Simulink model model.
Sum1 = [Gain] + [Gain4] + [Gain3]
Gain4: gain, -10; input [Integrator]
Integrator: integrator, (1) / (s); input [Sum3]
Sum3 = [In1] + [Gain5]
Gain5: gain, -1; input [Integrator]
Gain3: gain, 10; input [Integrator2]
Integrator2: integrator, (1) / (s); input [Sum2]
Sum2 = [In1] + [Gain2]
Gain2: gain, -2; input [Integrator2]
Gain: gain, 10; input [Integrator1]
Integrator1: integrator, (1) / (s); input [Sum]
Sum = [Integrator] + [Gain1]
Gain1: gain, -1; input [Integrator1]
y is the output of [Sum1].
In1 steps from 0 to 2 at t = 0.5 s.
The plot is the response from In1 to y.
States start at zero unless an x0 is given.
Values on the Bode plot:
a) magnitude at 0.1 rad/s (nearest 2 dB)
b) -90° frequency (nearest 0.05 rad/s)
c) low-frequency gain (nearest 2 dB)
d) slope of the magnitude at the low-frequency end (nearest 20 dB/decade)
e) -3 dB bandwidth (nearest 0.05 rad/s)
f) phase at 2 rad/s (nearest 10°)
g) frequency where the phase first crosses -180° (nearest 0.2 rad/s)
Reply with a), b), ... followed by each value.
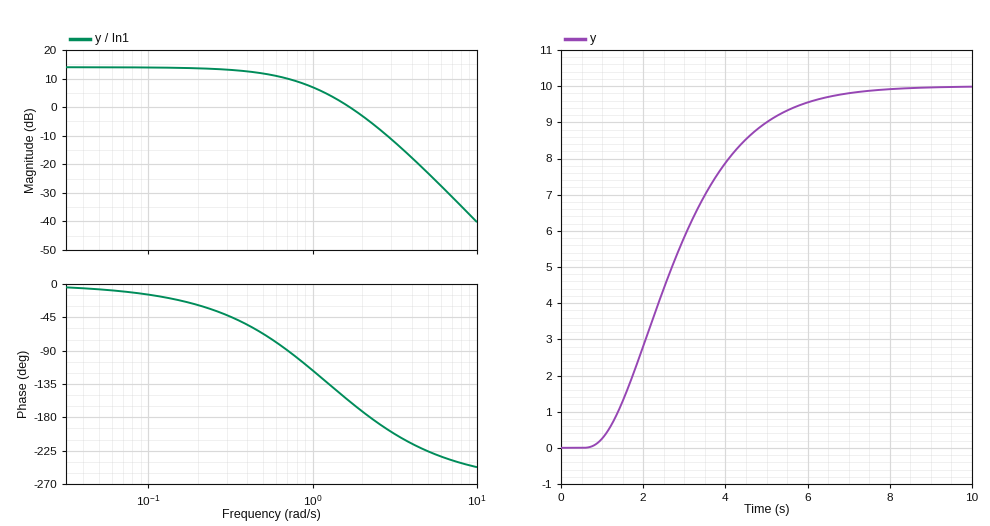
a) 14 dB
b) 0.70 rad/s
c) 14 dB
d) 0 dB/decade
e) 0.60 rad/s
f) -170°
g) 2.2 rad/s
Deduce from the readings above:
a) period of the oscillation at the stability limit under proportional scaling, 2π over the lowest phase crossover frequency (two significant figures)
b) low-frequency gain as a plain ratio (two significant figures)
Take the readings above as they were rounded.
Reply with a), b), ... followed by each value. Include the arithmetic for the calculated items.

a) 2π / 2.2 = 2.9 s
b) 10^(14 / 20) = 5.0
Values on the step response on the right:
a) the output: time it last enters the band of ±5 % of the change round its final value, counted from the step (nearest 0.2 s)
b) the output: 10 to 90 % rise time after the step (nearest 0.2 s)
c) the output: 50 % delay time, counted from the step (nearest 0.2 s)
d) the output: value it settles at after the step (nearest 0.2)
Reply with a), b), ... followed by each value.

a) 5.4 s
b) 3.6 s
c) 2.2 s
d) 10.0
